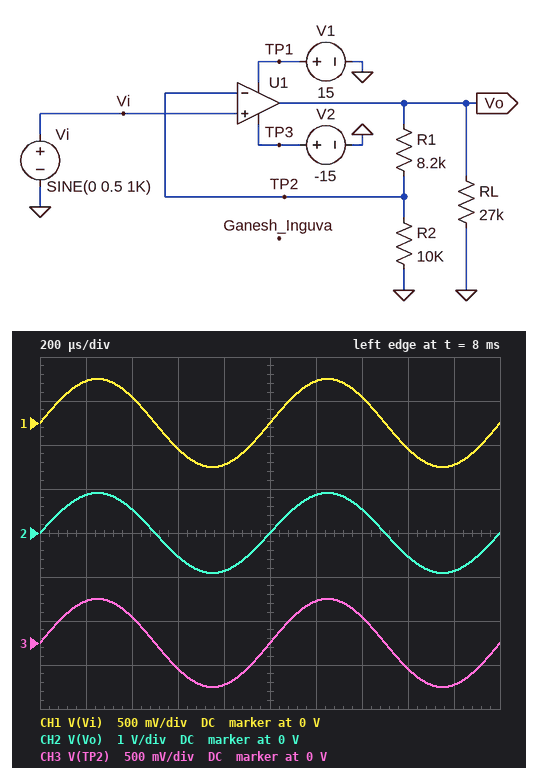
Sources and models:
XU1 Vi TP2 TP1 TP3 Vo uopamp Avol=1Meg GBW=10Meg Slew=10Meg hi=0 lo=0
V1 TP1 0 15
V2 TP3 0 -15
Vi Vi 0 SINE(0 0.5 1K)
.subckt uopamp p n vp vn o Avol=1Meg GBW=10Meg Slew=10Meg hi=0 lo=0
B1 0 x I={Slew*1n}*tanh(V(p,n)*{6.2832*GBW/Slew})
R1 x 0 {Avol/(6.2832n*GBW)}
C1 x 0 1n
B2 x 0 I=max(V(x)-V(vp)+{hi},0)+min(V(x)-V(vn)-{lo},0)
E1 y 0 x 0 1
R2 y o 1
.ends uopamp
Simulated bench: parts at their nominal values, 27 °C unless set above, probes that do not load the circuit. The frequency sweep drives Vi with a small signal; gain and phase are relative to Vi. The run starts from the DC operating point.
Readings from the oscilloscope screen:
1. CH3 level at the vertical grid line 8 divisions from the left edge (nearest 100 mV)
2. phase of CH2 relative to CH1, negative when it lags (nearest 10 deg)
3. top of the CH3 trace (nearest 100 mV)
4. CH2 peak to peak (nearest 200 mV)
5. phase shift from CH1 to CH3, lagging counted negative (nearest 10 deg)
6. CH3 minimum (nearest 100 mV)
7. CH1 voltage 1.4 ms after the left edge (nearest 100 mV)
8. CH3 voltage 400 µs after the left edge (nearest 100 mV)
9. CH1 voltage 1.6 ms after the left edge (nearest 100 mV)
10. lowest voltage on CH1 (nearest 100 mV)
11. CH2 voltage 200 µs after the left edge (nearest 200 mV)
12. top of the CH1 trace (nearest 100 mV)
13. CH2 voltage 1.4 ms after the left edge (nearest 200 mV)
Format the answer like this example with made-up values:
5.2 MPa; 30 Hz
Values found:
-300 mV; 0 deg; 500 mV; 1.8 V; 0 deg; -500 mV; 300 mV; 300 mV; -300 mV; -500 mV; 800 mV; 500 mV; 600 mV
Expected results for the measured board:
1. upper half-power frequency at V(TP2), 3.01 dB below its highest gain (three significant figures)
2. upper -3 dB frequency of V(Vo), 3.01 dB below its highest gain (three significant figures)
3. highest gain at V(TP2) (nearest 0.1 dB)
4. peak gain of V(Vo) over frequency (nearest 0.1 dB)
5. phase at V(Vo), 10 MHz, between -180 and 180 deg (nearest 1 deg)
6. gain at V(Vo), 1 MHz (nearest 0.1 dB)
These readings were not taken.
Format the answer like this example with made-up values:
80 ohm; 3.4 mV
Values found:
5.49 MHz; 5.49 MHz; 0 dB; 5.2 dB; -61 deg; 5.1 dB
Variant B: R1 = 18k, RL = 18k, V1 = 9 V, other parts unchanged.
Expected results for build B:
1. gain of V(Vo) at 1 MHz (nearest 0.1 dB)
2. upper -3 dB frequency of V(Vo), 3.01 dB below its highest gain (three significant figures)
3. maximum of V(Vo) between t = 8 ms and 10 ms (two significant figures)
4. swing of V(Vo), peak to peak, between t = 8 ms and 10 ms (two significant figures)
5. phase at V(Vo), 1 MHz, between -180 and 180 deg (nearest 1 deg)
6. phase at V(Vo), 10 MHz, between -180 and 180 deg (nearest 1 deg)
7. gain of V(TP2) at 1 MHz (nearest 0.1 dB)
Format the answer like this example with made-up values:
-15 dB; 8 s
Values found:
8.6 dB; 3.57 MHz; 1.4 V; 2.8 V; -16 deg; -70 deg; -0.3 dB
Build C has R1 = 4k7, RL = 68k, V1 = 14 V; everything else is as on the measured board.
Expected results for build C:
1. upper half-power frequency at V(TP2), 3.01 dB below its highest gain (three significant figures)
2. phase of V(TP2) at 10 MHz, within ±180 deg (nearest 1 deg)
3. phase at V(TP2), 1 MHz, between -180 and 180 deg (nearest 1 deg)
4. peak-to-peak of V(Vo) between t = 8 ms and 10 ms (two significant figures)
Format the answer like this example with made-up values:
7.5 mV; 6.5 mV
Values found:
6.80 MHz; -56 deg; -8 deg; 1.5 V
